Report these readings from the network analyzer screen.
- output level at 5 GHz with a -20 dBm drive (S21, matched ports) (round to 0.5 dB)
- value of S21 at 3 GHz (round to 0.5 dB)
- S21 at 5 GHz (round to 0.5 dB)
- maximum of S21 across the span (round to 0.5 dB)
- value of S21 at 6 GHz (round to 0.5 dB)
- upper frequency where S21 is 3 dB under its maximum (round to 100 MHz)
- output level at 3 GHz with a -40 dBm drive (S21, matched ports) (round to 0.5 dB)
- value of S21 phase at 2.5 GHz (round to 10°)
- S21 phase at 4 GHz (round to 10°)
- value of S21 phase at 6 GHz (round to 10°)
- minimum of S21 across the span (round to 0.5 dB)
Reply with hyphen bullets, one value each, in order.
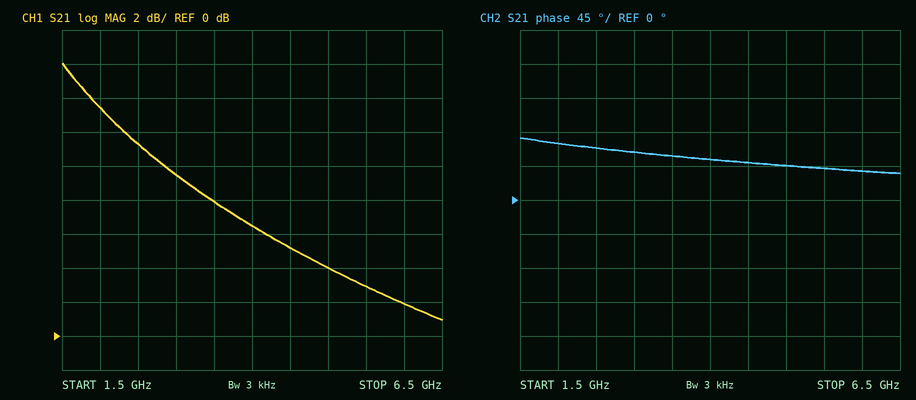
- -16.0 dBm
- 9.5 dB
- 4.0 dB
- 16.0 dB
- 2.0 dB
- 2.1 GHz
- -30.5 dBm
- 70°
- 50°
- 40°
- 1.0 dB
